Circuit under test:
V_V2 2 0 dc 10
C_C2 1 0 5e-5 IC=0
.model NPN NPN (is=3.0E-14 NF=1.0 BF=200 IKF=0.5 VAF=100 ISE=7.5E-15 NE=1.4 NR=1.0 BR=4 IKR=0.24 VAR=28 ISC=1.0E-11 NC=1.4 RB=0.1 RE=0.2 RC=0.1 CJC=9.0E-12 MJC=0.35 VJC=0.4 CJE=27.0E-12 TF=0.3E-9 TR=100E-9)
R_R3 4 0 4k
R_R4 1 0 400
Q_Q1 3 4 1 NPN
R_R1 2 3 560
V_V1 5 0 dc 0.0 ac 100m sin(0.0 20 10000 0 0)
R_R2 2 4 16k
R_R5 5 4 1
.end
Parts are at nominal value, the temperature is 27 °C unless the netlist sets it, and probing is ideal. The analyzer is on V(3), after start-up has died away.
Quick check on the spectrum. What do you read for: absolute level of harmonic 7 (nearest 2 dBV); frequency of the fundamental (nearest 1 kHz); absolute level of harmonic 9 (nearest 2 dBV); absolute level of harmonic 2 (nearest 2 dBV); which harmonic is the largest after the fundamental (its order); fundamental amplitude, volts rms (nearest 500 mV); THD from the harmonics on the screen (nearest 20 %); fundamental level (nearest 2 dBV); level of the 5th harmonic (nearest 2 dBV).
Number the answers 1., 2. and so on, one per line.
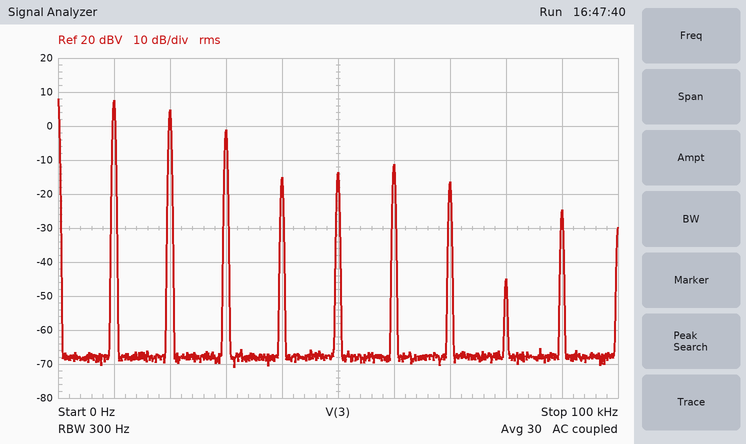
1. -16 dBV
2. 10 kHz
3. -24 dBV
4. 4 dBV
5. 2
6. 2.5 V
7. 80 %
8. 8 dBV
9. -14 dBV
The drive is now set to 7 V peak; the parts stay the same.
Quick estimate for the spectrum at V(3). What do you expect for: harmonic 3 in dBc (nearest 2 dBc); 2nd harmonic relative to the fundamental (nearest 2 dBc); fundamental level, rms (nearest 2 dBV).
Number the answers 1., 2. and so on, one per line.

1. -2 dBc
2. 0 dBc
3. -4 dBV
